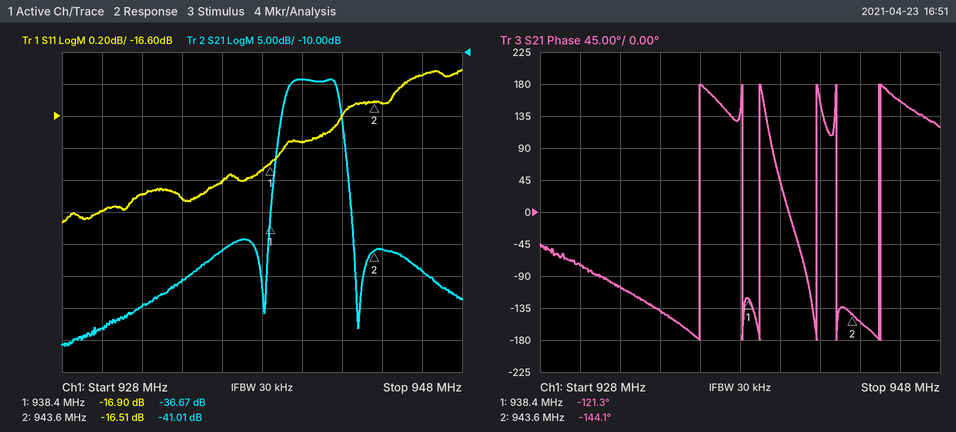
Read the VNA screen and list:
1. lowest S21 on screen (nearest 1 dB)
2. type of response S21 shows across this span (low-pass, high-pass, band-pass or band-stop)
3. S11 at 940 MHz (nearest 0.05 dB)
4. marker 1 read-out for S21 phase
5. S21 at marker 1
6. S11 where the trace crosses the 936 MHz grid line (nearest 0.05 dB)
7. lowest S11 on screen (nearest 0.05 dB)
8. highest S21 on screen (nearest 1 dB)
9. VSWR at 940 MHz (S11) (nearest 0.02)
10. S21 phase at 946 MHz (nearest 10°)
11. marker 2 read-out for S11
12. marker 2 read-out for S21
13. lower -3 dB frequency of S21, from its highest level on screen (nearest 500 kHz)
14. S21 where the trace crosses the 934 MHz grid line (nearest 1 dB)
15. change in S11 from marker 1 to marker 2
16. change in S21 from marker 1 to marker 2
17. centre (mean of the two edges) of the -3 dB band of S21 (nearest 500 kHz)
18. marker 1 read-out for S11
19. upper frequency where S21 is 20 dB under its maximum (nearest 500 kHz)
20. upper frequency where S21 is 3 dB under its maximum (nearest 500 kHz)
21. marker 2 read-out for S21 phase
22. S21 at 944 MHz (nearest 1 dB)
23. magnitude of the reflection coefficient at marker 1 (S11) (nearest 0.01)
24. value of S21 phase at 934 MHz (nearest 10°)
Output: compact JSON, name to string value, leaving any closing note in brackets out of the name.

{"lowest S21 on screen": "-56 dB", "type of response S21 shows across this span": "band-pass", "S11 at 940 MHz": "-16.75 dB", "marker 1 read-out for S21 phase": "-121.3°", "S21 at marker 1": "-36.67 dB", "S11 where the trace crosses the 936 MHz grid line": "-17.00 dB", "lowest S11 on screen": "-17.25 dB", "highest S21 on screen": "-14 dB", "VSWR at 940 MHz (S11)": "1.34", "S21 phase at 946 MHz": "160°", "marker 2 read-out for S11": "-16.51 dB", "marker 2 read-out for S21": "-41.01 dB", "lower -3 dB frequency of S21, from its highest level on screen": "939.0 MHz", "S21 where the trace crosses the 934 MHz grid line": "-46 dB", "change in S11 from marker 1 to marker 2": "0.39 dB", "change in S21 from marker 1 to marker 2": "-4.34 dB", "centre (mean of the two edges) of the -3 dB band of S21": "940.5 MHz", "marker 1 read-out for S11": "-16.90 dB", "upper frequency where S21 is 20 dB under its maximum": "942.5 MHz", "upper frequency where S21 is 3 dB under its maximum": "942.0 MHz", "marker 2 read-out for S21 phase": "-144.1°", "S21 at 944 MHz": "-41 dB", "magnitude of the reflection coefficient at marker 1 (S11)": "0.14", "value of S21 phase at 934 MHz": "-140°"}
